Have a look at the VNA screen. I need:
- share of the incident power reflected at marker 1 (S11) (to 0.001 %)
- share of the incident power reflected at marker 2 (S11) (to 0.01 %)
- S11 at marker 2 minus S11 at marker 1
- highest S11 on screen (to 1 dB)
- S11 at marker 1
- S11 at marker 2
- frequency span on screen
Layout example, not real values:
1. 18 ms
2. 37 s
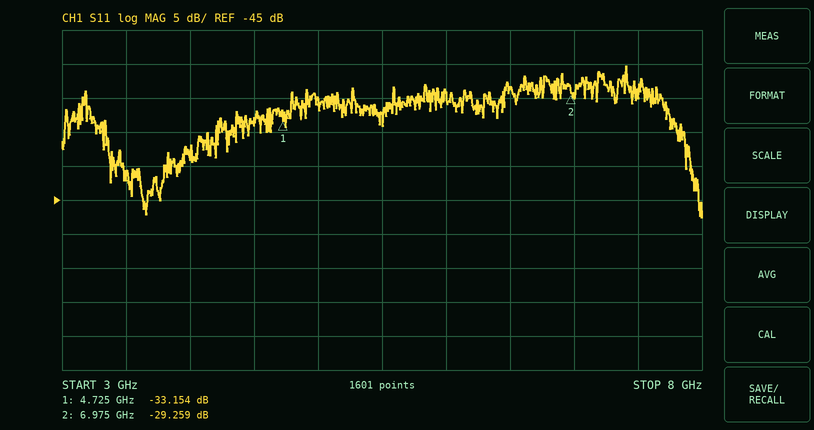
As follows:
1. 0.048 %
2. 0.12 %
3. 3.895 dB
4. -25 dB
5. -33.154 dB
6. -29.259 dB
7. 5 GHz
